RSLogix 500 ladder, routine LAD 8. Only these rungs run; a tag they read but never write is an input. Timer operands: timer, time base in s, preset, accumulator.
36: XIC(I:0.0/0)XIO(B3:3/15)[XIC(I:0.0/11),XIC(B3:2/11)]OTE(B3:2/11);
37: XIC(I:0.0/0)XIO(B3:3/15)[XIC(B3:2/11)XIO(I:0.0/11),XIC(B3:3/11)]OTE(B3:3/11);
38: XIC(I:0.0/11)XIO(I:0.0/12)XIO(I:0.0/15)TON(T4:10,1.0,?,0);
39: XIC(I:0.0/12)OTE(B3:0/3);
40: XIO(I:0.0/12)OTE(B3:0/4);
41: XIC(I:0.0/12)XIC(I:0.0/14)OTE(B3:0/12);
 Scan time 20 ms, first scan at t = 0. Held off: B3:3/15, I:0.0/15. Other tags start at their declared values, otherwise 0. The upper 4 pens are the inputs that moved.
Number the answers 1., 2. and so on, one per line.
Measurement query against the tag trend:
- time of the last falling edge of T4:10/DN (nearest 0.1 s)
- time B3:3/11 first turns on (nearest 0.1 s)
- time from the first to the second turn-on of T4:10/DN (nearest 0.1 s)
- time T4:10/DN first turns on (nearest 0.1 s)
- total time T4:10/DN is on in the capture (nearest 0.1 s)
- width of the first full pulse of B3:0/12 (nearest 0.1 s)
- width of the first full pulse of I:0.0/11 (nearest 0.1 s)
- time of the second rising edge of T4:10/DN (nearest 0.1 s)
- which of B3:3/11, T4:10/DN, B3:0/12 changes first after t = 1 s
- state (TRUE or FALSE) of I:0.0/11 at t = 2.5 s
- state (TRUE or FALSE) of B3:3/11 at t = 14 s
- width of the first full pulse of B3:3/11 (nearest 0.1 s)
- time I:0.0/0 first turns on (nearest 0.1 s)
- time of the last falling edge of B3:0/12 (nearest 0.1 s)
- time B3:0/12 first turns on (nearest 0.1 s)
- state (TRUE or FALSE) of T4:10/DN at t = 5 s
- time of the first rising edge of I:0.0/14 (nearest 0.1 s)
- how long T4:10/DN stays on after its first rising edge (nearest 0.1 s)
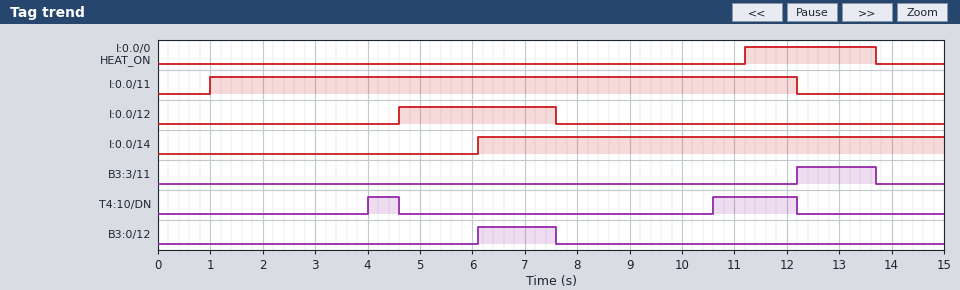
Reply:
1. 12.2 s
2. 12.2 s
3. 6.6 s
4. 4.0 s
5. 2.2 s
6. 1.5 s
7. 11.2 s
8. 10.6 s
9. T4:10/DN
10. TRUE
11. FALSE
12. 1.5 s
13. 11.2 s
14. 7.6 s
15. 6.1 s
16. FALSE
17. 6.1 s
18. 0.6 s
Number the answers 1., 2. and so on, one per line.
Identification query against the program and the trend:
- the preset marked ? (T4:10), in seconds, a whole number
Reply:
1. 3 s
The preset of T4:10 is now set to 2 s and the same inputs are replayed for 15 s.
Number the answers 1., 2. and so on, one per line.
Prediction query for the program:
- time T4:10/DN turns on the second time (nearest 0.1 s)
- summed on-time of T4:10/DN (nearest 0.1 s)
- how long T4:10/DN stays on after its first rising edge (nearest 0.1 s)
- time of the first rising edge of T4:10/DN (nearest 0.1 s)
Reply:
1. 9.6 s
2. 4.2 s
3. 1.6 s
4. 3.0 s
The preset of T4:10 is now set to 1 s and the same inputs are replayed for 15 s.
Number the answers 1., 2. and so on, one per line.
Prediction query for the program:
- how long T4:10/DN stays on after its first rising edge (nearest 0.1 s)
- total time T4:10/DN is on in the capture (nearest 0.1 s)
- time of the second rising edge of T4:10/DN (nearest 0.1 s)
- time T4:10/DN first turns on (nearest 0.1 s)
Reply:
1. 2.6 s
2. 6.2 s
3. 8.6 s
4. 2.0 s
